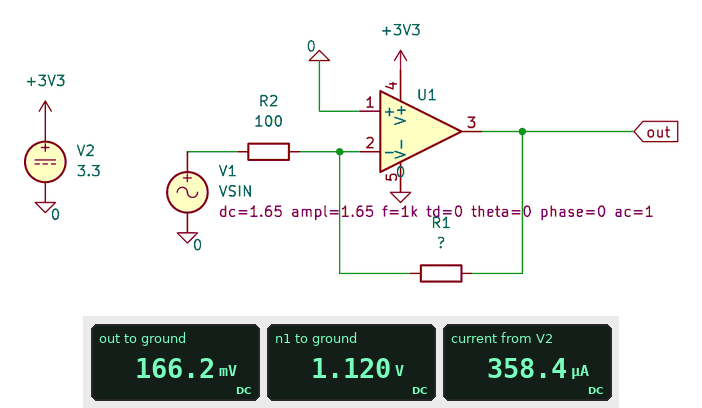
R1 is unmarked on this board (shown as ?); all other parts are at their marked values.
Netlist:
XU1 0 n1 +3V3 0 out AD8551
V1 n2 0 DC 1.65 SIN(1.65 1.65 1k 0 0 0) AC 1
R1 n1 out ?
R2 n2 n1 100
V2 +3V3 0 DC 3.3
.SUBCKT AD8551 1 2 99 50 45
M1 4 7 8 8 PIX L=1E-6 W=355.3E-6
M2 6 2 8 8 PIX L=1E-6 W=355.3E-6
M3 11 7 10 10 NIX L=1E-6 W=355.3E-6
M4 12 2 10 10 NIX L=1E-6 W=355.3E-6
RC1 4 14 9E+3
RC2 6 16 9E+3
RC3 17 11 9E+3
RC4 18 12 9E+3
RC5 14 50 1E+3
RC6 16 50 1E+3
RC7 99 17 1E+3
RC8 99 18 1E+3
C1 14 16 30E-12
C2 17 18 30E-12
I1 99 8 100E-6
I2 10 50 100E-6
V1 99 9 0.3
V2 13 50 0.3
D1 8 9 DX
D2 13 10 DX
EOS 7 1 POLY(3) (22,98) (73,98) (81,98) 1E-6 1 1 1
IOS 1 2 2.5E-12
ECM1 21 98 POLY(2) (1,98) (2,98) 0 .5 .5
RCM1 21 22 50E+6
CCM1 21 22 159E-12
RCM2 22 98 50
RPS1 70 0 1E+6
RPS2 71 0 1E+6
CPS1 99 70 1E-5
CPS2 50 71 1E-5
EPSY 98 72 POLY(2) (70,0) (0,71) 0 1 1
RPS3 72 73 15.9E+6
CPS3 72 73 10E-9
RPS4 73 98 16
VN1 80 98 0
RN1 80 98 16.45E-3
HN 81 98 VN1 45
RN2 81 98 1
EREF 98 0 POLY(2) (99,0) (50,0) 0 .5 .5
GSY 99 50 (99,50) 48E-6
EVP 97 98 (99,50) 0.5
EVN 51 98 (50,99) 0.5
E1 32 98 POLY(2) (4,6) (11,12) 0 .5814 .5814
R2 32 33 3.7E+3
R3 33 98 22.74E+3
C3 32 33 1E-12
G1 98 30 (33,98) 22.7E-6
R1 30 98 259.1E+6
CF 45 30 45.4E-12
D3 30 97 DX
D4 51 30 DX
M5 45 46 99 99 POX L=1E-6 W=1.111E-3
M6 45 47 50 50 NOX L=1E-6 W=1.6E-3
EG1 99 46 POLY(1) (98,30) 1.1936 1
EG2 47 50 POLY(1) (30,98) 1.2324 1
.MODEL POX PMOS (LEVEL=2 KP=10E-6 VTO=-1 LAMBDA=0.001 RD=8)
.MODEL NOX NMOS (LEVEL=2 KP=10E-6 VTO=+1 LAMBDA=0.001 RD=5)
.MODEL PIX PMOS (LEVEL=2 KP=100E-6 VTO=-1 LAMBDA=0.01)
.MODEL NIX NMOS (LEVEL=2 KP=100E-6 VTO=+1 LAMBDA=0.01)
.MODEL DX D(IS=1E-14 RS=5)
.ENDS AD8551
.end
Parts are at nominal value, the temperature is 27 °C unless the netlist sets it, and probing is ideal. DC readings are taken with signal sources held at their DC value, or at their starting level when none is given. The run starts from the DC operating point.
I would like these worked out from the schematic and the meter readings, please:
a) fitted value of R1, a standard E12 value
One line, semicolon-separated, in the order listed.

180 Ω
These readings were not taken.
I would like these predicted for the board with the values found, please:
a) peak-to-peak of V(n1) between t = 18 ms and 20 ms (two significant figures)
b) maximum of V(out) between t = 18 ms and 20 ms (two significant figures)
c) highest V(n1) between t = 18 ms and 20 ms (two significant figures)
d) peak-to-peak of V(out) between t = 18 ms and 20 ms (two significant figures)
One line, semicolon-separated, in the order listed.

2.2 V; 340 mV; 2.2 V; 340 mV
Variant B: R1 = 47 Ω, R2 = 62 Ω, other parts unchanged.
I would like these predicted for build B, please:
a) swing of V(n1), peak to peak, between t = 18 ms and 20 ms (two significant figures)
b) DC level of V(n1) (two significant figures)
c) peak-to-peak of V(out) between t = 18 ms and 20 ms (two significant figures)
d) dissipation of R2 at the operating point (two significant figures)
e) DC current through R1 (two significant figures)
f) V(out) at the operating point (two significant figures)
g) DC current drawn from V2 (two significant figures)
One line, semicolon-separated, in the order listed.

1.9 V; 930 mV; 800 mV; 8.4 mW; 12 mA; 380 mV; 360 µA
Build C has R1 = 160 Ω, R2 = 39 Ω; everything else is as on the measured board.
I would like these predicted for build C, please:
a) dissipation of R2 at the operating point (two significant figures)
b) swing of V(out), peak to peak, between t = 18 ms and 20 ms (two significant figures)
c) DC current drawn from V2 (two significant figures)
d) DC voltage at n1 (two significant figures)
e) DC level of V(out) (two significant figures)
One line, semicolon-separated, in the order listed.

2.0 mW; 470 mV; 360 µA; 1.4 V; 230 mV
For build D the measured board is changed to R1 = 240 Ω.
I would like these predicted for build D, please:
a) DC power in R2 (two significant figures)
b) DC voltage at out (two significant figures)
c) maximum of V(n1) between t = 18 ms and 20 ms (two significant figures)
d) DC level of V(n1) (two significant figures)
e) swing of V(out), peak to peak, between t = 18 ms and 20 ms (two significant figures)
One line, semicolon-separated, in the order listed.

2.0 mW; 140 mV; 2.4 V; 1.2 V; 280 mV
